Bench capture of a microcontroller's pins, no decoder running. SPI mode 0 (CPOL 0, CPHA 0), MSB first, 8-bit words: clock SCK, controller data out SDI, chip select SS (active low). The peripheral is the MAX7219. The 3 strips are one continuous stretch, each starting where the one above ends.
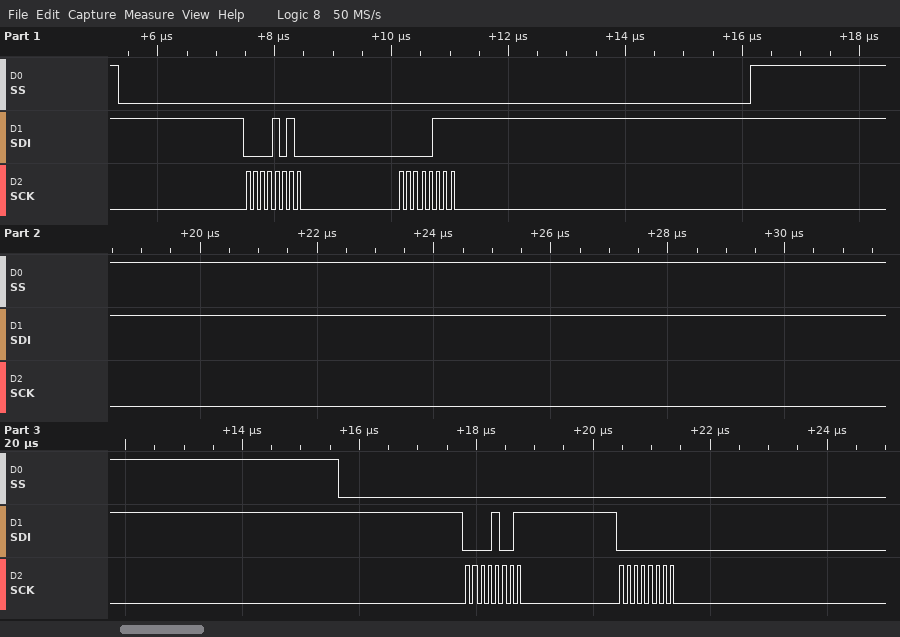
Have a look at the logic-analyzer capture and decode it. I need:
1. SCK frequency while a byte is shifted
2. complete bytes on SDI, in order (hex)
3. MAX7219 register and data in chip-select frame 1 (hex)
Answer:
8 MHz
0A 07 09 00
register 0xA, data 0x07
